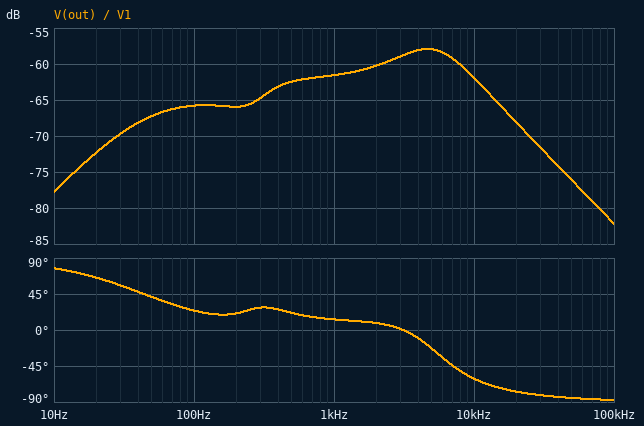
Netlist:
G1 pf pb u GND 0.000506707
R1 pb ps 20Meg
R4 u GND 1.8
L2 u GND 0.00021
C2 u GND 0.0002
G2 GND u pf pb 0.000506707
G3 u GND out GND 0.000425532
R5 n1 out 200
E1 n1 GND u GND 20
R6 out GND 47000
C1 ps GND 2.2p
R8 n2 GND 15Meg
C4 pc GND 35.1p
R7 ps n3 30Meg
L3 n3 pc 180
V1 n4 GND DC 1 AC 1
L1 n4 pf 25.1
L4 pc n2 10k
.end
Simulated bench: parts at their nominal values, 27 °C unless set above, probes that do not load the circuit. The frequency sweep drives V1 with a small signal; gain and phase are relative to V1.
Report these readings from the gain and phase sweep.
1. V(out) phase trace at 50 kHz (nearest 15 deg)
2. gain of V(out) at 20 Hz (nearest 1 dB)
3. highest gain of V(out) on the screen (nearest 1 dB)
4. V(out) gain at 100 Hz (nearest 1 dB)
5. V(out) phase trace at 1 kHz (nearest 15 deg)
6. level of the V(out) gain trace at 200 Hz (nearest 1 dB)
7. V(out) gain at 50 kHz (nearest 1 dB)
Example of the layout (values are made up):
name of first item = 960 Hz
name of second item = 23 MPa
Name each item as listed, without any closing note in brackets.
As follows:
V(out) phase trace at 50 kHz = -90 deg
gain of V(out) at 20 Hz = -72 dB
highest gain of V(out) on the screen = -58 dB
V(out) gain at 100 Hz = -66 dB
V(out) phase trace at 1 kHz = 15 deg
level of the V(out) gain trace at 200 Hz = -66 dB
V(out) gain at 50 kHz = -76 dB
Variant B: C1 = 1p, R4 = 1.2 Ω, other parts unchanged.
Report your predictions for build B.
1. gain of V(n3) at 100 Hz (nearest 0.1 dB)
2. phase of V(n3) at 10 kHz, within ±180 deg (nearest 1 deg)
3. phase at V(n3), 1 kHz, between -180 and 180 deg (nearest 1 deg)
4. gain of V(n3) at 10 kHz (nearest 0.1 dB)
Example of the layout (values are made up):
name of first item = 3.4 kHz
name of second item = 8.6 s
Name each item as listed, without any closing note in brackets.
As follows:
gain of V(n3) at 100 Hz = -12.8 dB
phase of V(n3) at 10 kHz, within ±180 deg = -39 deg
phase at V(n3), 1 kHz, between -180 and 180 deg = -92 deg
gain of V(n3) at 10 kHz = -18.5 dB
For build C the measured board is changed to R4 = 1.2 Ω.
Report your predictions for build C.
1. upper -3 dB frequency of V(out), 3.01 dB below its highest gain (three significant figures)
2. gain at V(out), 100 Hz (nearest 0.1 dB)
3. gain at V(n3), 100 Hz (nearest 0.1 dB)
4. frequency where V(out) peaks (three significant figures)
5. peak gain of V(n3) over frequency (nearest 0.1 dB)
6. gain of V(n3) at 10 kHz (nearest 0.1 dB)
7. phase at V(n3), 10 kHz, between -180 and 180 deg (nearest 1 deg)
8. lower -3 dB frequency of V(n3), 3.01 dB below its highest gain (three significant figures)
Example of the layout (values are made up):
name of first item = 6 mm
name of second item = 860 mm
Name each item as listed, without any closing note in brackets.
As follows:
upper -3 dB frequency of V(out), 3.01 dB below its highest gain = 9.06 kHz
gain at V(out), 100 Hz = -65.9 dB
gain at V(n3), 100 Hz = -12.9 dB
frequency where V(out) peaks = 4.71 kHz
peak gain of V(n3) over frequency = -9.9 dB
gain of V(n3) at 10 kHz = -25.6 dB
phase at V(n3), 10 kHz, between -180 and 180 deg = -67 deg
lower -3 dB frequency of V(n3), 3.01 dB below its highest gain = 99.2 Hz
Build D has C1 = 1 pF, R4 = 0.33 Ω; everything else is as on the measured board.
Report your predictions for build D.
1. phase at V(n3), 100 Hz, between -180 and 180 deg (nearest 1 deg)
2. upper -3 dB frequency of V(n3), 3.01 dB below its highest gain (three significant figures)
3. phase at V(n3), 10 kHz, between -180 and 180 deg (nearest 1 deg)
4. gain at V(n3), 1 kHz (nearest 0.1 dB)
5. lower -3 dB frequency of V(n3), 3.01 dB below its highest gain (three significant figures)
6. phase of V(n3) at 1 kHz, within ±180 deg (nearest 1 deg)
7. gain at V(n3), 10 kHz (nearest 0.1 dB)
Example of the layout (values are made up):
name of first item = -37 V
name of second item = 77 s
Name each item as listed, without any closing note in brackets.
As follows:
phase at V(n3), 100 Hz, between -180 and 180 deg = 21 deg
upper -3 dB frequency of V(n3), 3.01 dB below its highest gain = 427 Hz
phase at V(n3), 10 kHz, between -180 and 180 deg = -32 deg
gain at V(n3), 1 kHz = -24.5 dB
lower -3 dB frequency of V(n3), 3.01 dB below its highest gain = 100 Hz
phase of V(n3) at 1 kHz, within ±180 deg = -93 deg
gain at V(n3), 10 kHz = -19.5 dB
